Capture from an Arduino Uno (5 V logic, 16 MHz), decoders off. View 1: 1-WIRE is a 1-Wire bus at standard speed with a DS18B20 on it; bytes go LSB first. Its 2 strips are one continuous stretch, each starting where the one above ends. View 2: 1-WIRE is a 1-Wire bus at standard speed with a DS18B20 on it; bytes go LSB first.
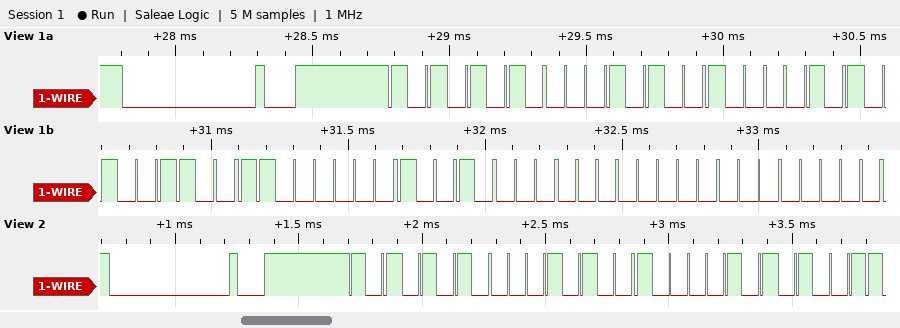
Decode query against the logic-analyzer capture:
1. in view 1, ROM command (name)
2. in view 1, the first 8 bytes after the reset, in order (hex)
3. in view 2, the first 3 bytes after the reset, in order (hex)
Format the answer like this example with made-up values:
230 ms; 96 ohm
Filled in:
Match ROM; 55 28 A1 32 03 09 00 00; 55 28 A1
